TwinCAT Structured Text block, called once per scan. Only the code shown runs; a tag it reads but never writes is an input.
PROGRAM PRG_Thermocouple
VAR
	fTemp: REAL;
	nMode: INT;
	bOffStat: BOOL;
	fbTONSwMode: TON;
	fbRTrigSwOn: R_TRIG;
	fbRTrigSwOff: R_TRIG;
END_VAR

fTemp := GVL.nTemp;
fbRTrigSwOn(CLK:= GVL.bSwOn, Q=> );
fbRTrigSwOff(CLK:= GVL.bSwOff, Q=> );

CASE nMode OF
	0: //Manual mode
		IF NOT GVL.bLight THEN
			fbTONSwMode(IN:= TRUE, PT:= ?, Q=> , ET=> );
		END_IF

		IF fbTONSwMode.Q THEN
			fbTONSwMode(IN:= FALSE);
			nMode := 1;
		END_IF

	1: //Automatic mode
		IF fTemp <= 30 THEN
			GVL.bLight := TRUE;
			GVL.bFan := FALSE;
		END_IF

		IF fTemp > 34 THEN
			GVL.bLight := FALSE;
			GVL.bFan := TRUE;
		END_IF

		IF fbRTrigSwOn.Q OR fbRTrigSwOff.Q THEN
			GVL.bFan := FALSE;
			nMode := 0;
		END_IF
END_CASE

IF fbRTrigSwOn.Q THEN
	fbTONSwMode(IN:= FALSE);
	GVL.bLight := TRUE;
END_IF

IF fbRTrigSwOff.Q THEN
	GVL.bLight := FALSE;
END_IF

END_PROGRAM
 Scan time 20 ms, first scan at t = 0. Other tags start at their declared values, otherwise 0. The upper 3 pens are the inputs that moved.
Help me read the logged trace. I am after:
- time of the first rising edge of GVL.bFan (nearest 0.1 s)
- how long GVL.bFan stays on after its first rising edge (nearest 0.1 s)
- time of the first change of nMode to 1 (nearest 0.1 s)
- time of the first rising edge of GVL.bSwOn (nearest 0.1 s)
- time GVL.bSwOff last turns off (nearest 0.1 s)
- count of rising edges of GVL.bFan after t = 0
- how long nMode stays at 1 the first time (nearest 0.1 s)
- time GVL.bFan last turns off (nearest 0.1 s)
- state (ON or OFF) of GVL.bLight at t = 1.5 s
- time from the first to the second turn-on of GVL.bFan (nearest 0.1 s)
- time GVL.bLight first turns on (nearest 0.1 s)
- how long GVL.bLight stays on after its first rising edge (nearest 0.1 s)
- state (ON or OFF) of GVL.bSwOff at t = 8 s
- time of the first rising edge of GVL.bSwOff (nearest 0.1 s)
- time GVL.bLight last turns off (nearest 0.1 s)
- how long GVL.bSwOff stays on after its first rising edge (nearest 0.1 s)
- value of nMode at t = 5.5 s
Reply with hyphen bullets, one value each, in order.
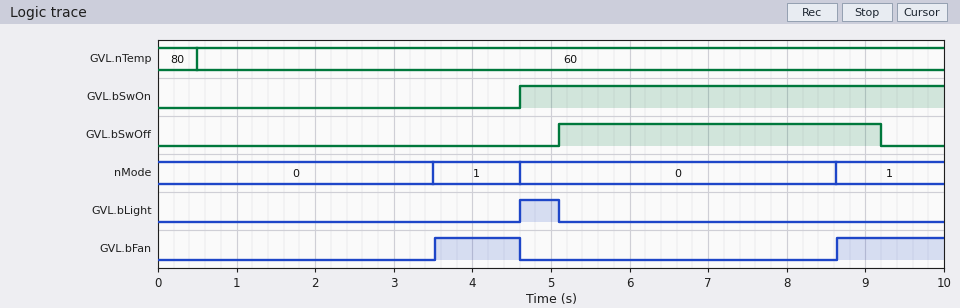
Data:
- 3.5 s
- 1.1 s
- 3.5 s
- 4.6 s
- 9.2 s
- 2
- 1.1 s
- 4.6 s
- OFF
- 5.1 s
- 4.6 s
- 0.5 s
- ON
- 5.1 s
- 5.1 s
- 4.1 s
- 0
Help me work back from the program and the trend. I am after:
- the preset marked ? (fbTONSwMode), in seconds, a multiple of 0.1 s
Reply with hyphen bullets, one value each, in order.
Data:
- 3.5 s
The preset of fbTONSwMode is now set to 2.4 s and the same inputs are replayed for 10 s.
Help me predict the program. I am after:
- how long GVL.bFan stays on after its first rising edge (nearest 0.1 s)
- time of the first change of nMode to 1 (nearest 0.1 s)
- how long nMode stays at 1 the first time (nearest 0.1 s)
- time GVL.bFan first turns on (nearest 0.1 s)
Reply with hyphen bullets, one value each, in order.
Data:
- 2.2 s
- 2.4 s
- 2.2 s
- 2.4 s
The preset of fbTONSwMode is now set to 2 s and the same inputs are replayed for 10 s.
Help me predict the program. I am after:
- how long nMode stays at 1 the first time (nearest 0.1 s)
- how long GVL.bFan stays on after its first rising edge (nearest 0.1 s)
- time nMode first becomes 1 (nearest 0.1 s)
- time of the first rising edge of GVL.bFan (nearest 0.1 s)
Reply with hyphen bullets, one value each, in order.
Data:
- 2.6 s
- 2.6 s
- 2.0 s
- 2.0 s
